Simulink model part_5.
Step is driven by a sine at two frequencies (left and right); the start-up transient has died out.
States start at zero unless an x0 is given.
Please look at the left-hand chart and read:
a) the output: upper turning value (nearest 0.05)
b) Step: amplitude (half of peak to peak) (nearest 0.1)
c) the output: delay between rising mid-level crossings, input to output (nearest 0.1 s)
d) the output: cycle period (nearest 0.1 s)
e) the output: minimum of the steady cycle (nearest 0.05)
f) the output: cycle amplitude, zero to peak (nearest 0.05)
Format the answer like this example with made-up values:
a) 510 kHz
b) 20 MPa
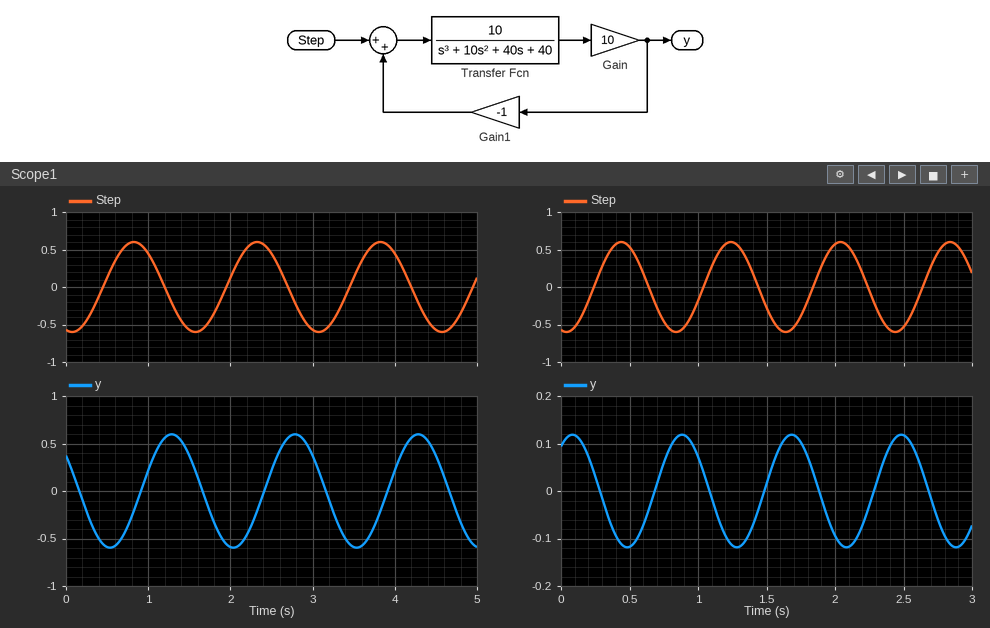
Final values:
a) 0.60
b) 0.6
c) 0.5 s
d) 1.5 s
e) -0.60
f) 0.60
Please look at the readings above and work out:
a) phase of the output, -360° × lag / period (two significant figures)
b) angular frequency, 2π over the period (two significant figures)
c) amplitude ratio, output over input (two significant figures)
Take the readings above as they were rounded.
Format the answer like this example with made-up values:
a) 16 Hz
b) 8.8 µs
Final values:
a) -120°
b) 4.2 rad/s
c) 1.0
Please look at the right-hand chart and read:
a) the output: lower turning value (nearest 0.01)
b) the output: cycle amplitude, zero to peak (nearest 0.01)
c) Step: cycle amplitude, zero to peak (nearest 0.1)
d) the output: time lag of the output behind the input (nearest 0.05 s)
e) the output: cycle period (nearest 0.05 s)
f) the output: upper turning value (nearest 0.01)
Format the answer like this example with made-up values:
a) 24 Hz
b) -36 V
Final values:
a) -0.12
b) 0.12
c) 0.6
d) 0.45 s
e) 0.80 s
f) 0.12
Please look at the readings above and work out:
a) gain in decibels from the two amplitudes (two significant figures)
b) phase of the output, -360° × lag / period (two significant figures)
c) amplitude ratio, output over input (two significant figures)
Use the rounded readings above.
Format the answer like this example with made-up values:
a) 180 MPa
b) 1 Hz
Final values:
a) -14 dB
b) -200°
c) 0.20
